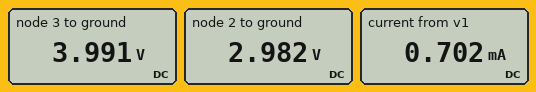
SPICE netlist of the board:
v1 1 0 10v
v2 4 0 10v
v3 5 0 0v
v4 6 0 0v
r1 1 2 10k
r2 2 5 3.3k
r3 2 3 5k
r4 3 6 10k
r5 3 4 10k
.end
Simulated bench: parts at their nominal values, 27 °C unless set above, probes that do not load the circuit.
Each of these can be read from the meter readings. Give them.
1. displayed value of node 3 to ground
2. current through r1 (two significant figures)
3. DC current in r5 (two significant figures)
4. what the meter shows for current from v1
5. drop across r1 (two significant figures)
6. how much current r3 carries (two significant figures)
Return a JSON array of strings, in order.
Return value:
["3.991 V", "700 µA", "600 µA", "0.702 mA", "7.0 V", "200 µA"]
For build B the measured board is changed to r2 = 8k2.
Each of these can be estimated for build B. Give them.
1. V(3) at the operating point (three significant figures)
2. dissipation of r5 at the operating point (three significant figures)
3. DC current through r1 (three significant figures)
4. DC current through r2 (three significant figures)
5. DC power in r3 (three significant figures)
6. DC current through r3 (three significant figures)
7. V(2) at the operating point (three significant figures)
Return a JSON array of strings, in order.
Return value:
["4.83 V", "2.67 mW", "534 µA", "568 µA", "5.81 µW", "34.1 µA", "4.66 V"]
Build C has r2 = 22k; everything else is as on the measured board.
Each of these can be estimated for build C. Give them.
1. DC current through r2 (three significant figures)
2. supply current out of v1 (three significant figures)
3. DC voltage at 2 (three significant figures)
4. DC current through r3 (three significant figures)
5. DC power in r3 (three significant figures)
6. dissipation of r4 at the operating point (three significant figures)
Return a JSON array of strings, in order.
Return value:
["278 µA", "389 µA", "6.11 V", "111 µA", "61.7 µW", "3.09 mW"]
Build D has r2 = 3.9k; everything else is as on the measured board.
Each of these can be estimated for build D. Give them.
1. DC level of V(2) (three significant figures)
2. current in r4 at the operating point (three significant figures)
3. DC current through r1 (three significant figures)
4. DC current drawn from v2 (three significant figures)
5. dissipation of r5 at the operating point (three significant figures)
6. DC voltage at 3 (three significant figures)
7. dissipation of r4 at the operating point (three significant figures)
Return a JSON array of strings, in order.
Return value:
["3.29 V", "414 µA", "671 µA", "586 µA", "3.43 mW", "4.14 V", "1.72 mW"]
